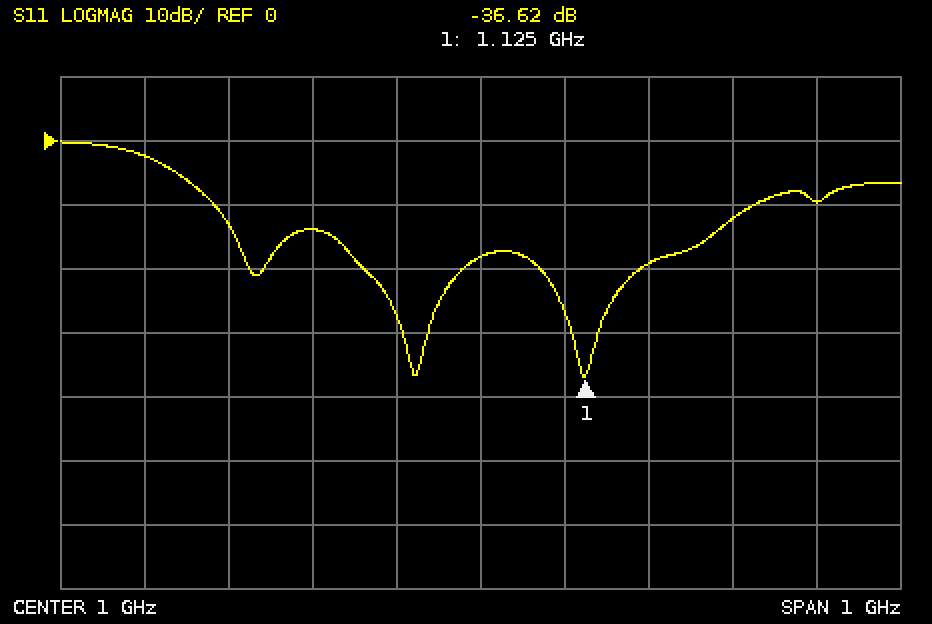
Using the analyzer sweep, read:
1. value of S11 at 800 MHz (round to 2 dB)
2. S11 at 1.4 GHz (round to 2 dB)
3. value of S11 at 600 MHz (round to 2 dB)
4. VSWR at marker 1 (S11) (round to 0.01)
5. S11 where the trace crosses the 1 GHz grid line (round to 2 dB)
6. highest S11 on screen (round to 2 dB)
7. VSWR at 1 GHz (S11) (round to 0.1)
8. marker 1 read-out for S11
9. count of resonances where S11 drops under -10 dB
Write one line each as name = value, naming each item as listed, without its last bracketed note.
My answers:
value of S11 at 800 MHz = -14 dB
S11 at 1.4 GHz = -10 dB
value of S11 at 600 MHz = -2 dB
VSWR at marker 1 (S11) = 1.03
S11 where the trace crosses the 1 GHz grid line = -18 dB
highest S11 on screen = 0 dB
VSWR at 1 GHz (S11) = 1.3
marker 1 read-out for S11 = -36.62 dB
count of resonances where S11 drops under -10 dB = 3
